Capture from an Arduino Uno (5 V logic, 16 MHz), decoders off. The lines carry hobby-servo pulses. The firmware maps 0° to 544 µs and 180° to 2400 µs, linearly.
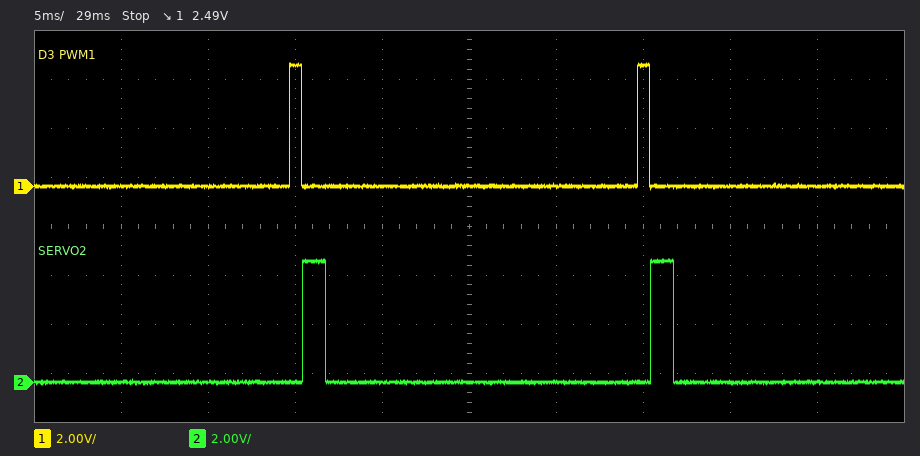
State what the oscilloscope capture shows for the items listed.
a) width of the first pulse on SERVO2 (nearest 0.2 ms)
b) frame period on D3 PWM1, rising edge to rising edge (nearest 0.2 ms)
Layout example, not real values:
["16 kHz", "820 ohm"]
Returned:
["1.4 ms", "20.0 ms"]
